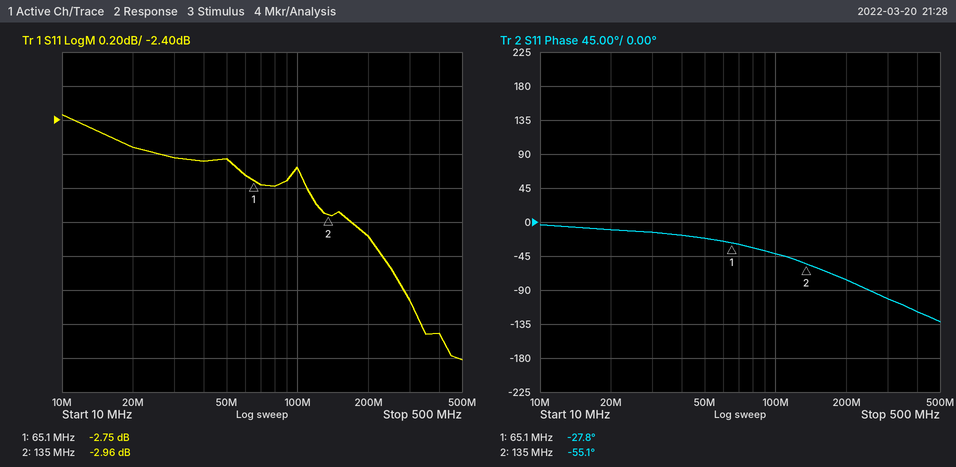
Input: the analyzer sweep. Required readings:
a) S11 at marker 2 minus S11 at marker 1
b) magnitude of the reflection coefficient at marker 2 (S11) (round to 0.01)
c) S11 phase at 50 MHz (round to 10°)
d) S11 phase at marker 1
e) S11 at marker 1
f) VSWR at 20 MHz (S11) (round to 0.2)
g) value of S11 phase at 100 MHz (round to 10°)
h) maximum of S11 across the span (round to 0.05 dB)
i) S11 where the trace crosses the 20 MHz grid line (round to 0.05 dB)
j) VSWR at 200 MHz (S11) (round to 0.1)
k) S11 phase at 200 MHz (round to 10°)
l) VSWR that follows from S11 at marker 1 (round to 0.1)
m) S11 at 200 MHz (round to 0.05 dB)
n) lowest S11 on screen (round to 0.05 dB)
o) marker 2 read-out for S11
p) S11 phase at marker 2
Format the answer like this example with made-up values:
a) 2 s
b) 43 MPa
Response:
a) -0.21 dB
b) 0.71
c) -20°
d) -27.8°
e) -2.75 dB
f) 6.8
g) -40°
h) -2.35 dB
i) -2.55 dB
j) 5.7
k) -80°
l) 6.4
m) -3.10 dB
n) -3.80 dB
o) -2.96 dB
p) -55.1°
